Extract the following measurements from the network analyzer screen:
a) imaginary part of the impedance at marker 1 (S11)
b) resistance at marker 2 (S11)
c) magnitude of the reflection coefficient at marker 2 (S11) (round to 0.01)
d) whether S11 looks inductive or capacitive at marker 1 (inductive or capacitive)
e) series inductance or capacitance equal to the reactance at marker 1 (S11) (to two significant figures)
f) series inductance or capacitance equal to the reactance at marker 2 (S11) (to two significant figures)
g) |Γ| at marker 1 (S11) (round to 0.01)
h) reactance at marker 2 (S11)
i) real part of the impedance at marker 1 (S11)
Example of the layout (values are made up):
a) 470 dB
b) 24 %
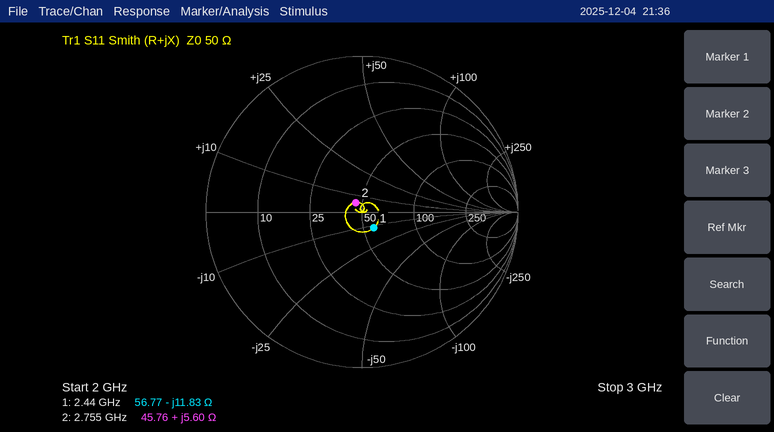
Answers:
a) -11.83 Ω
b) 45.76 Ω
c) 0.07
d) capacitive
e) 5.5 pF
f) 320 pH
g) 0.13
h) +5.60 Ω
i) 56.77 Ω
